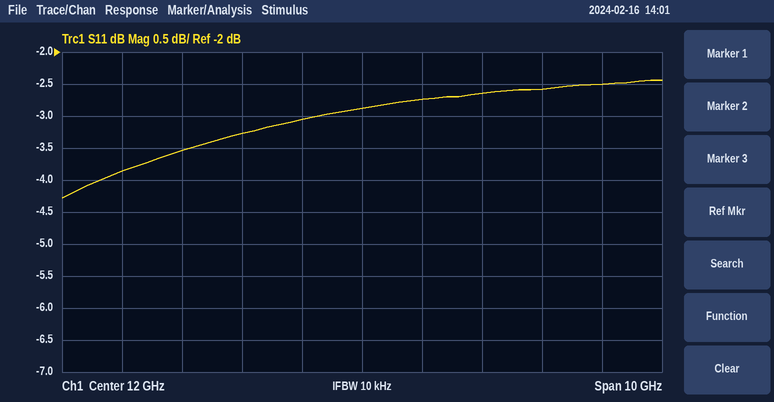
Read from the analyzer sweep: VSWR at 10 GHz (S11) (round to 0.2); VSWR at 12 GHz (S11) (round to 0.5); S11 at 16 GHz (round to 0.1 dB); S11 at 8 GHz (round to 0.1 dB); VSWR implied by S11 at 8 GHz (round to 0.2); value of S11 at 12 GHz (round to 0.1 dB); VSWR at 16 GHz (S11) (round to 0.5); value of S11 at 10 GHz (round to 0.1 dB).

5.4
6.0
-2.5 dB
-3.9 dB
4.6
-2.9 dB
7.0
-3.3 dB
